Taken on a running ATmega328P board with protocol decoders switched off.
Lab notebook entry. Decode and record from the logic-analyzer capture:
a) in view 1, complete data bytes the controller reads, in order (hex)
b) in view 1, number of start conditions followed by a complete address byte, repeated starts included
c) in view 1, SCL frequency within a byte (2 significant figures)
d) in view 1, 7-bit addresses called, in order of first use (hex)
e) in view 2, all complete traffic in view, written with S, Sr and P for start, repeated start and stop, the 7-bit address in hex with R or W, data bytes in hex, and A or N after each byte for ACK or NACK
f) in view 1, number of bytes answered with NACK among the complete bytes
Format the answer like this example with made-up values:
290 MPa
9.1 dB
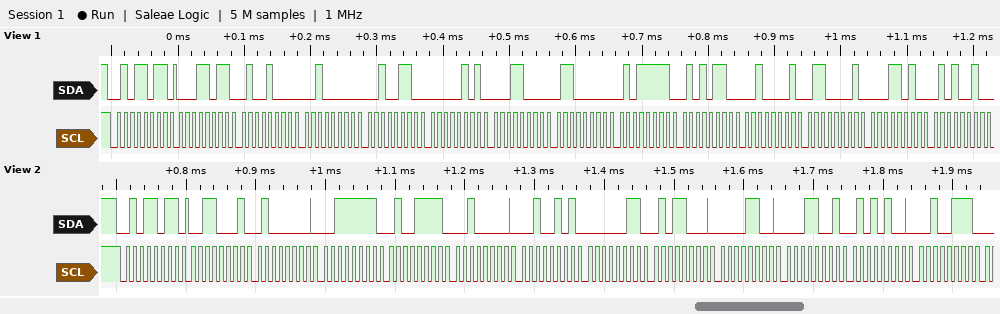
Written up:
1B 48 20 26 05 18 60 5F 56 21 61 1A 52
1
100 kHz
0x2D
S 2DR A 31 A 40 A 3F A 4F A 20 A 25 A 03 A 58 A 0C A 19 A 54 A 27 A
0
